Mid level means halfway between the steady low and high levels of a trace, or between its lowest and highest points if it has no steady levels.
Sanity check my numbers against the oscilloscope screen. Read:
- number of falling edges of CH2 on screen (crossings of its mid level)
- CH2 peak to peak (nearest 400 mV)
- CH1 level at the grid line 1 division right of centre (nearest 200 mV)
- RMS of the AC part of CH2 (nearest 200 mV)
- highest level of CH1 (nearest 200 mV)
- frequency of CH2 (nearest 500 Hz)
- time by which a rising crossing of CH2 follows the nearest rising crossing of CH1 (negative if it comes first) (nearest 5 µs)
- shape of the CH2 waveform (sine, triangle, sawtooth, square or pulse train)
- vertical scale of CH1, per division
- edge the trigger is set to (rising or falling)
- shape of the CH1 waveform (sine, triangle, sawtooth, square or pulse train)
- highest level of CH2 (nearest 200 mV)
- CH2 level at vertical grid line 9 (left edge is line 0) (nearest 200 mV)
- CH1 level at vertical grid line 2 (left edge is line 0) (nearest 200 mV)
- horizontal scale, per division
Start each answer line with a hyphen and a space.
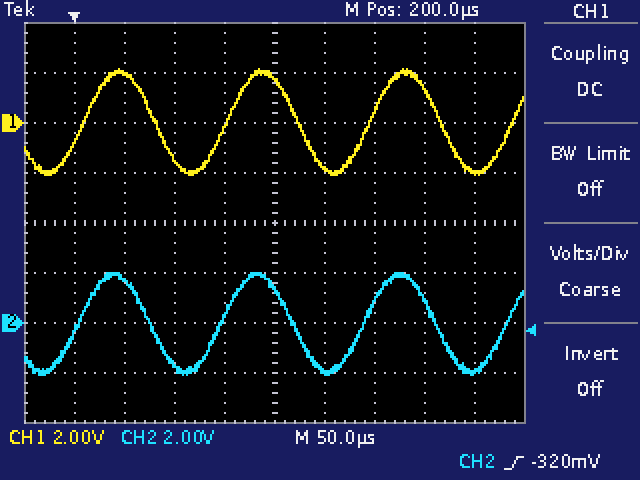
- 3
- 4.0 V
- -1.8 V
- 1.4 V
- 2.2 V
- 7.0 kHz
- -5 µs
- sine
- 2 V
- rising
- sine
- 2.0 V
- -2.0 V
- 2.0 V
- 50 µs
